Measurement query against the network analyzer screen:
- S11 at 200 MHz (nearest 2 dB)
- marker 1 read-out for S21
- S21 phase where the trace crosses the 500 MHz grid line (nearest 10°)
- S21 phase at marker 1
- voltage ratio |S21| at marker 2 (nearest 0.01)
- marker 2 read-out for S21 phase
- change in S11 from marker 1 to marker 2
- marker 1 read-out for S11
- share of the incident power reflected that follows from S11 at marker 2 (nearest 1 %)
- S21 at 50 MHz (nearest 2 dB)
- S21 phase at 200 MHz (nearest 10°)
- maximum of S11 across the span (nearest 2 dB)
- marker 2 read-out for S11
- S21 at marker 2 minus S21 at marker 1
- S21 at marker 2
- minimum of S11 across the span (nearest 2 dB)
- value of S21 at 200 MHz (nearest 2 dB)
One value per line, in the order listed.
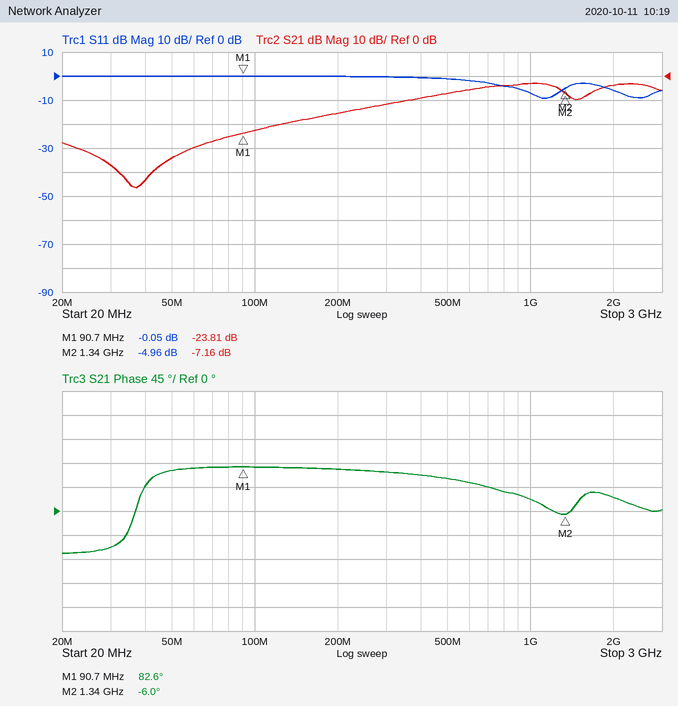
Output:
0 dB
-23.81 dB
60°
82.6°
0.44
-6.0°
-4.91 dB
-0.05 dB
32 %
-34 dB
80°
0 dB
-4.96 dB
16.65 dB
-7.16 dB
-10 dB
-16 dB
